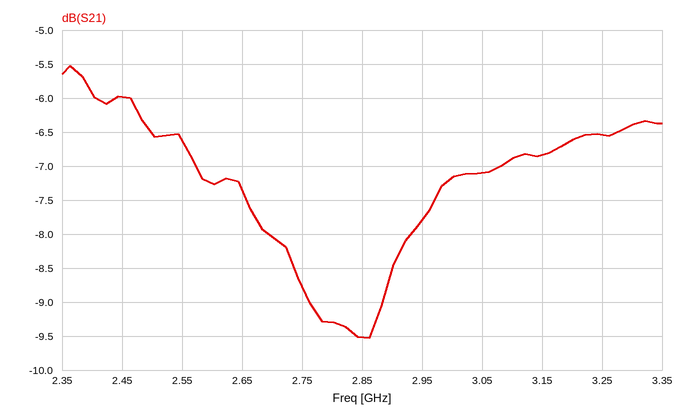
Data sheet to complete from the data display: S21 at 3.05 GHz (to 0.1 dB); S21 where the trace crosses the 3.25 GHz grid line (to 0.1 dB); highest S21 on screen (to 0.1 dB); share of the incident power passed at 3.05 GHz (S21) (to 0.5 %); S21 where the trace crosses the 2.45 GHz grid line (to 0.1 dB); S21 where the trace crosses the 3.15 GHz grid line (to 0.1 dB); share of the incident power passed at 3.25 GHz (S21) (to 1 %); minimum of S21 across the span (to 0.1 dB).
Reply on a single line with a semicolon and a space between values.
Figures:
-7.1 dB; -6.5 dB; -5.5 dB; 19.5 %; -6.0 dB; -6.8 dB; 22 %; -9.5 dB
